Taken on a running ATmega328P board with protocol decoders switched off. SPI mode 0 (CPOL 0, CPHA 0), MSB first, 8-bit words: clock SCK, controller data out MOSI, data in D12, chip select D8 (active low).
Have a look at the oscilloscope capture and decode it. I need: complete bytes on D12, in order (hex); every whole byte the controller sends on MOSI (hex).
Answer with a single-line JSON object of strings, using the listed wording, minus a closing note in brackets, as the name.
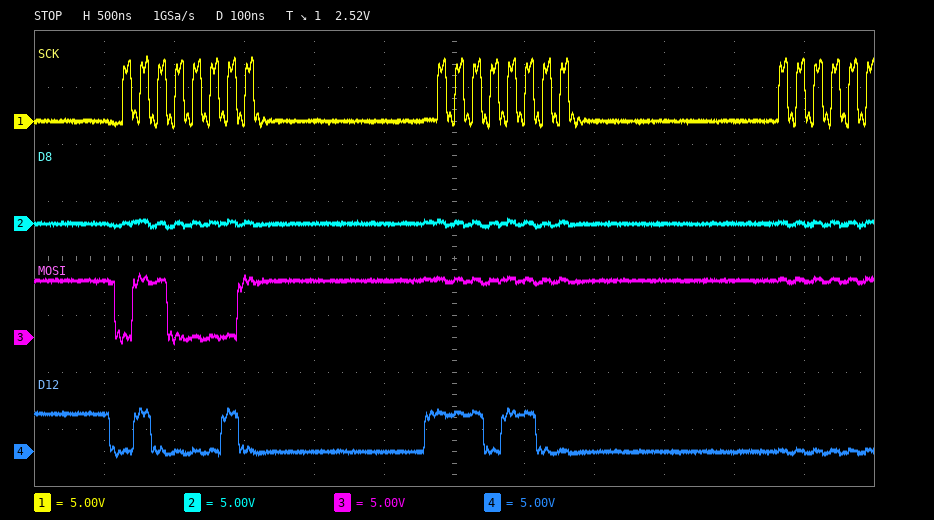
{"complete bytes on D12, in order": "42 EC", "every whole byte the controller sends on MOSI": "61 FF"}
